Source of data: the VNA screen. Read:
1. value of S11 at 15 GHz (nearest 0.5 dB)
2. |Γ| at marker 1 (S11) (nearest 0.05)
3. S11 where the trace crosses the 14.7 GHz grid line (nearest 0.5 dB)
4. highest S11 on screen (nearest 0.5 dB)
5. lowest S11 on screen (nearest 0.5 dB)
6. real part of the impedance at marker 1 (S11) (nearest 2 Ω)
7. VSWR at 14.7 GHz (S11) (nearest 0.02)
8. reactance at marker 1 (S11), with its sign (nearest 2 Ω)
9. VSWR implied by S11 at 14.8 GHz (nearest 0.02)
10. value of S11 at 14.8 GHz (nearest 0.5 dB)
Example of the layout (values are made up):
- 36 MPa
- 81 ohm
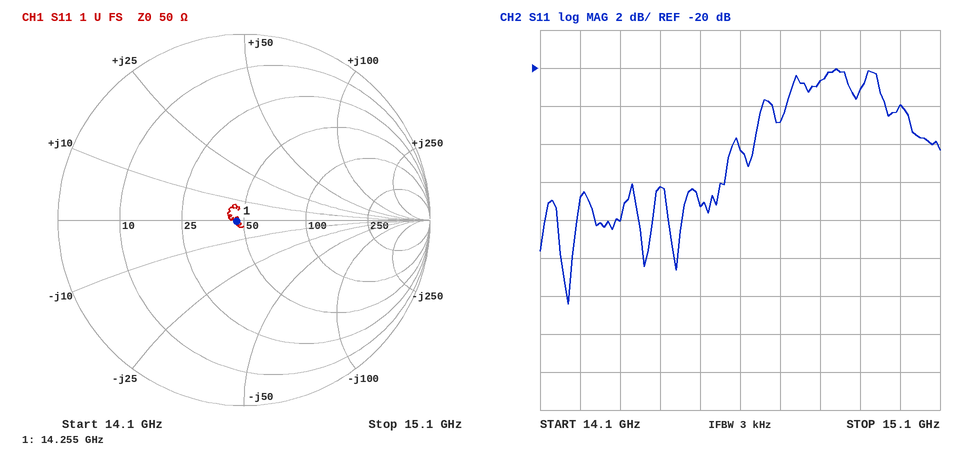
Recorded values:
- -22.0 dB
- 0.05
- -23.0 dB
- -20.0 dB
- -32.5 dB
- 46 Ω
- 1.16
- 0 Ω
- 1.20
- -20.5 dB
